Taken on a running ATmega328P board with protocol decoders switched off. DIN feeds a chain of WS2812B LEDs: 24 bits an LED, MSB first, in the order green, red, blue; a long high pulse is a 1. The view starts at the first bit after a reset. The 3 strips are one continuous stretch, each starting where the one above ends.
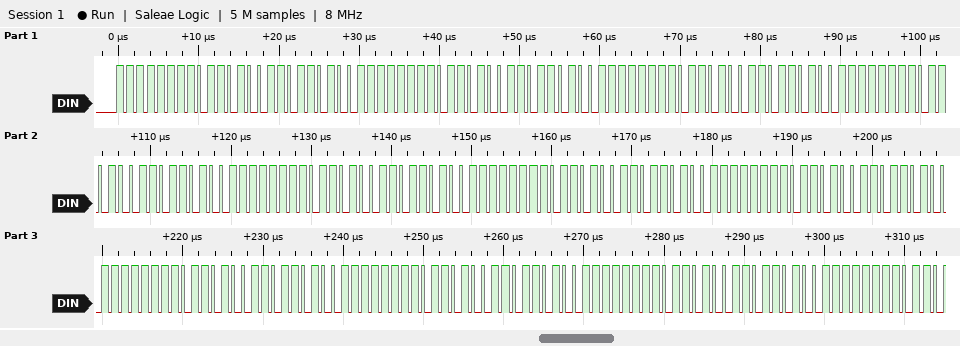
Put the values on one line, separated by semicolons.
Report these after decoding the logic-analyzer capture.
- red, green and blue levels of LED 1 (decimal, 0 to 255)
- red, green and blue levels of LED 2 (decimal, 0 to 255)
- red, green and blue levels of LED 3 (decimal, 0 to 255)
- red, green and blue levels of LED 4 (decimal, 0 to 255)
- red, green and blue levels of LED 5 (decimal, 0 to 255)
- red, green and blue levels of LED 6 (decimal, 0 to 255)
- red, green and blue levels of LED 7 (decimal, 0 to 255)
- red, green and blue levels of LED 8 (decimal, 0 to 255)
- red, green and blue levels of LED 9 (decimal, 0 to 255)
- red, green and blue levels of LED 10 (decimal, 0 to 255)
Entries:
105, 255, 180; 105, 255, 180; 105, 255, 180; 105, 255, 180; 105, 255, 180; 105, 255, 180; 105, 255, 180; 105, 255, 180; 105, 255, 180; 105, 255, 180
